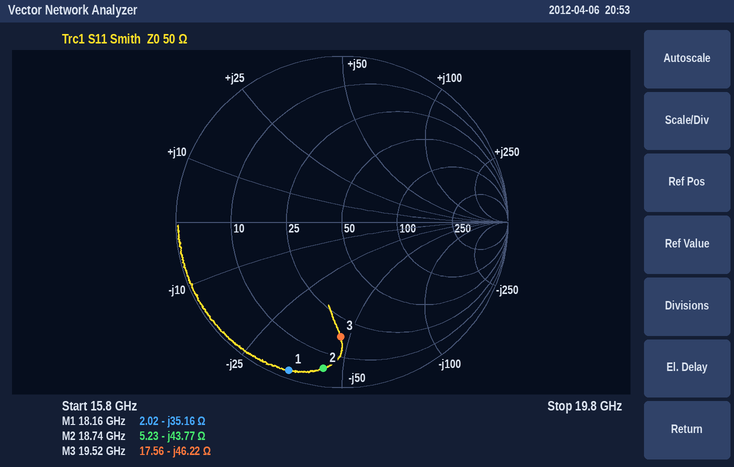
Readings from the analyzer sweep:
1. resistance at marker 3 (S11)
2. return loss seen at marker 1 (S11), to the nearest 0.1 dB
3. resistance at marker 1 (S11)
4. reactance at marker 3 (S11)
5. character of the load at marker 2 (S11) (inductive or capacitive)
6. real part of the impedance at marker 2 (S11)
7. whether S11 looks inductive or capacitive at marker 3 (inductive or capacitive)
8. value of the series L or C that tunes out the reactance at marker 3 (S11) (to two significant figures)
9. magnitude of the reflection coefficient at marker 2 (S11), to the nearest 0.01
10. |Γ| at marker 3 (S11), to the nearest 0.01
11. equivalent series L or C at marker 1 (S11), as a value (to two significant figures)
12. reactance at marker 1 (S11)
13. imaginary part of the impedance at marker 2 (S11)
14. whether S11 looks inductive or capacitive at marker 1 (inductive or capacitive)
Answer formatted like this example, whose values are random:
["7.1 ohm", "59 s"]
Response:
["17.56 Ω", "0.5 dB", "2.02 Ω", "-46.22 Ω", "capacitive", "5.23 Ω", "capacitive", "380 pH", "0.89", "0.69", "250 fF", "-35.16 Ω", "-43.77 Ω", "capacitive"]
